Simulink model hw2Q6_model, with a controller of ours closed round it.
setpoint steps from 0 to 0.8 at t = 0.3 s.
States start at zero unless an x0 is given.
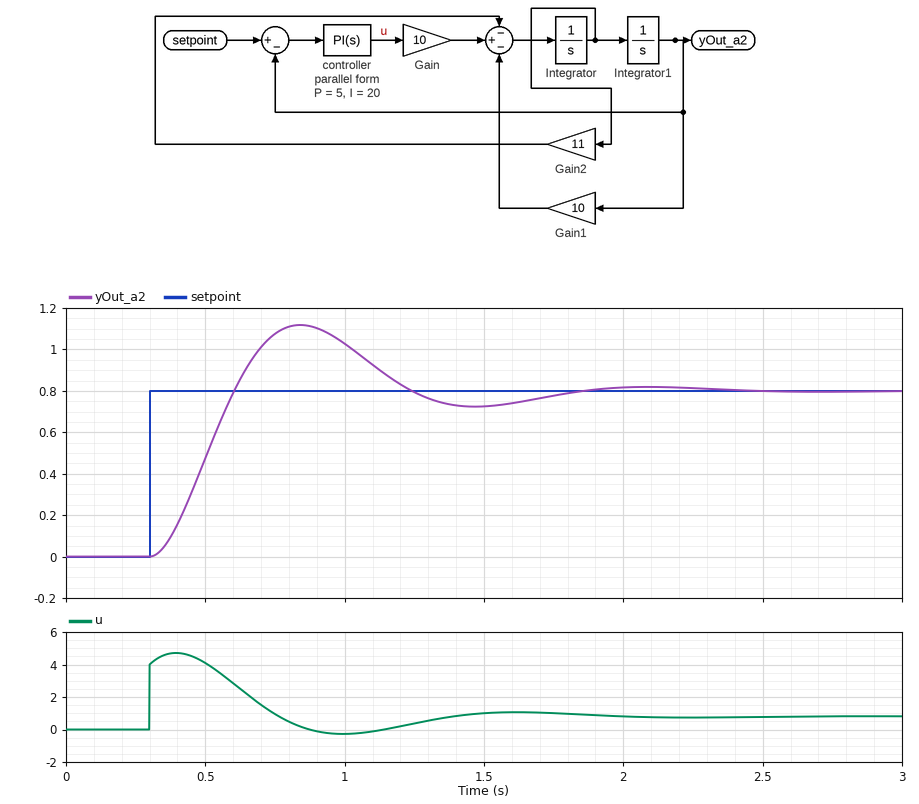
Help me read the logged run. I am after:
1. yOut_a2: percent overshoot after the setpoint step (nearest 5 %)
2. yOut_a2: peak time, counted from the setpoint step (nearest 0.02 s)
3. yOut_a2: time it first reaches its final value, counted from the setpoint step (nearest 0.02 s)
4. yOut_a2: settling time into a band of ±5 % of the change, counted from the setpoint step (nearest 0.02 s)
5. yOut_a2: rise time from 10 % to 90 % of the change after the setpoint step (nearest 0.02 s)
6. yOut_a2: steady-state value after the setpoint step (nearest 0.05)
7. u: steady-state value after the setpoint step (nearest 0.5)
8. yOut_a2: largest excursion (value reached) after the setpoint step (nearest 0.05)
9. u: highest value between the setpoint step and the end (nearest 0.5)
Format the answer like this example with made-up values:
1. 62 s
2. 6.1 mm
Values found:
1. 40 %
2. 0.54 s
3. 0.30 s
4. 1.38 s
5. 0.20 s
6. 0.80
7. 1.0
8. 1.10
9. 4.5
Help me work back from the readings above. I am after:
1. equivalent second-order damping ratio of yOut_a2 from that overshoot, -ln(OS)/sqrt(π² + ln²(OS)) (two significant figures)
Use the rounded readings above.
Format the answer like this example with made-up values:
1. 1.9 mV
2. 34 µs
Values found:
1. 0.28
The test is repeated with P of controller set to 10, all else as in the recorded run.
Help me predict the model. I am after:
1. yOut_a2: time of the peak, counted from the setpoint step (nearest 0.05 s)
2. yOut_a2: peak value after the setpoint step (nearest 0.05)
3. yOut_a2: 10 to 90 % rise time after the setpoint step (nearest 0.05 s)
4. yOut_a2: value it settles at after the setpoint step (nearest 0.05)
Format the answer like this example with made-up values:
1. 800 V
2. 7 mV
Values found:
1. 0.35 s
2. 1.00
3. 0.15 s
4. 0.80
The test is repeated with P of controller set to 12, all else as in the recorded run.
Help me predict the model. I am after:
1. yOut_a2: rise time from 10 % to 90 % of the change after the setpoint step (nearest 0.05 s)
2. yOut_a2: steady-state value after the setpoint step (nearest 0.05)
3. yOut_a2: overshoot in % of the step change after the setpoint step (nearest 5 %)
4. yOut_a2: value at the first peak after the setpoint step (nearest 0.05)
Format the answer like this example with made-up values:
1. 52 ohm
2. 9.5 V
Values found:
1. 0.15 s
2. 0.80
3. 25 %
4. 1.00
